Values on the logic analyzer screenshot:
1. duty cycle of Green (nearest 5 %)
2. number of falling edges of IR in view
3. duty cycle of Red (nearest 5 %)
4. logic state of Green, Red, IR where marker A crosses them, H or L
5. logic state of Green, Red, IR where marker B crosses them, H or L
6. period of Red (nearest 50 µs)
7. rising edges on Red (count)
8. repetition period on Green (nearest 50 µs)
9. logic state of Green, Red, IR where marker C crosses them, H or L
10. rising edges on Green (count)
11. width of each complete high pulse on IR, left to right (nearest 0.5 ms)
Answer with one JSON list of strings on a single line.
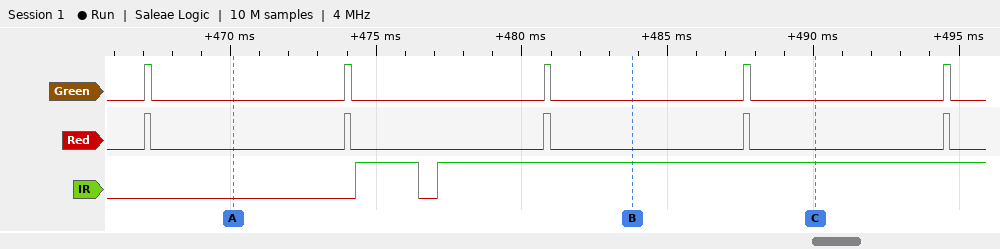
["5 %", "1", "5 %", "Green=L, Red=L, IR=L", "Green=L, Red=L, IR=H", "6850 µs", "5", "6850 µs", "Green=L, Red=L, IR=H", "5", "2 ms"]
